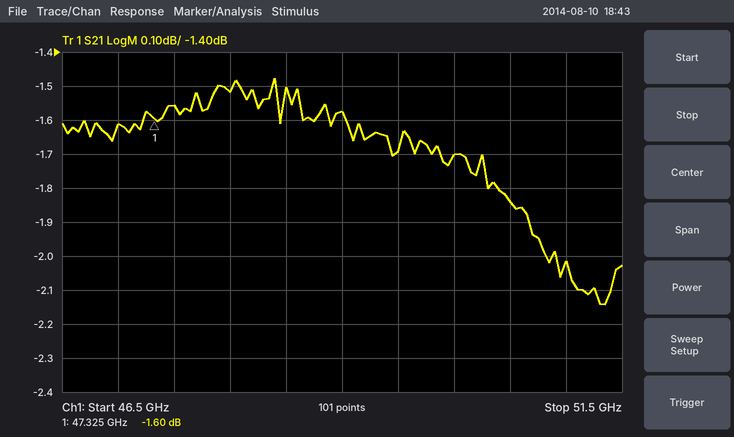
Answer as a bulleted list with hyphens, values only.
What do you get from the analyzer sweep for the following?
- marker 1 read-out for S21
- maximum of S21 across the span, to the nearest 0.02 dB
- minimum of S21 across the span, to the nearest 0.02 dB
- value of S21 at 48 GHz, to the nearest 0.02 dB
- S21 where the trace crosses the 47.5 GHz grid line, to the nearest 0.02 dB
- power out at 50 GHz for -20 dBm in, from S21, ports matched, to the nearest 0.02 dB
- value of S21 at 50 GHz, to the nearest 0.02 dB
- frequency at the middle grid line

- -1.60 dB
- -1.48 dB
- -2.14 dB
- -1.52 dB
- -1.56 dB
- -21.70 dBm
- -1.70 dB
- 49 GHz
